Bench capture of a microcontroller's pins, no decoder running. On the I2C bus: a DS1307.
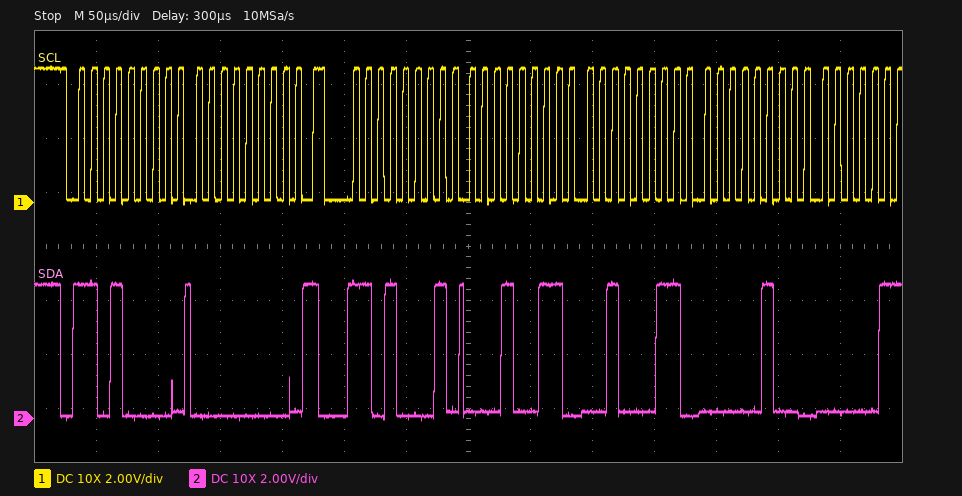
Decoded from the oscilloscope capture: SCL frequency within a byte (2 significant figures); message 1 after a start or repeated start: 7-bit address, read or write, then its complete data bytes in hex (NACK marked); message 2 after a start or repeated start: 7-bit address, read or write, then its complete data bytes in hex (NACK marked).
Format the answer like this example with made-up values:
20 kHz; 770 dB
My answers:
100 kHz; 0x68 write: 00; 0x68 read: 13 23 04
